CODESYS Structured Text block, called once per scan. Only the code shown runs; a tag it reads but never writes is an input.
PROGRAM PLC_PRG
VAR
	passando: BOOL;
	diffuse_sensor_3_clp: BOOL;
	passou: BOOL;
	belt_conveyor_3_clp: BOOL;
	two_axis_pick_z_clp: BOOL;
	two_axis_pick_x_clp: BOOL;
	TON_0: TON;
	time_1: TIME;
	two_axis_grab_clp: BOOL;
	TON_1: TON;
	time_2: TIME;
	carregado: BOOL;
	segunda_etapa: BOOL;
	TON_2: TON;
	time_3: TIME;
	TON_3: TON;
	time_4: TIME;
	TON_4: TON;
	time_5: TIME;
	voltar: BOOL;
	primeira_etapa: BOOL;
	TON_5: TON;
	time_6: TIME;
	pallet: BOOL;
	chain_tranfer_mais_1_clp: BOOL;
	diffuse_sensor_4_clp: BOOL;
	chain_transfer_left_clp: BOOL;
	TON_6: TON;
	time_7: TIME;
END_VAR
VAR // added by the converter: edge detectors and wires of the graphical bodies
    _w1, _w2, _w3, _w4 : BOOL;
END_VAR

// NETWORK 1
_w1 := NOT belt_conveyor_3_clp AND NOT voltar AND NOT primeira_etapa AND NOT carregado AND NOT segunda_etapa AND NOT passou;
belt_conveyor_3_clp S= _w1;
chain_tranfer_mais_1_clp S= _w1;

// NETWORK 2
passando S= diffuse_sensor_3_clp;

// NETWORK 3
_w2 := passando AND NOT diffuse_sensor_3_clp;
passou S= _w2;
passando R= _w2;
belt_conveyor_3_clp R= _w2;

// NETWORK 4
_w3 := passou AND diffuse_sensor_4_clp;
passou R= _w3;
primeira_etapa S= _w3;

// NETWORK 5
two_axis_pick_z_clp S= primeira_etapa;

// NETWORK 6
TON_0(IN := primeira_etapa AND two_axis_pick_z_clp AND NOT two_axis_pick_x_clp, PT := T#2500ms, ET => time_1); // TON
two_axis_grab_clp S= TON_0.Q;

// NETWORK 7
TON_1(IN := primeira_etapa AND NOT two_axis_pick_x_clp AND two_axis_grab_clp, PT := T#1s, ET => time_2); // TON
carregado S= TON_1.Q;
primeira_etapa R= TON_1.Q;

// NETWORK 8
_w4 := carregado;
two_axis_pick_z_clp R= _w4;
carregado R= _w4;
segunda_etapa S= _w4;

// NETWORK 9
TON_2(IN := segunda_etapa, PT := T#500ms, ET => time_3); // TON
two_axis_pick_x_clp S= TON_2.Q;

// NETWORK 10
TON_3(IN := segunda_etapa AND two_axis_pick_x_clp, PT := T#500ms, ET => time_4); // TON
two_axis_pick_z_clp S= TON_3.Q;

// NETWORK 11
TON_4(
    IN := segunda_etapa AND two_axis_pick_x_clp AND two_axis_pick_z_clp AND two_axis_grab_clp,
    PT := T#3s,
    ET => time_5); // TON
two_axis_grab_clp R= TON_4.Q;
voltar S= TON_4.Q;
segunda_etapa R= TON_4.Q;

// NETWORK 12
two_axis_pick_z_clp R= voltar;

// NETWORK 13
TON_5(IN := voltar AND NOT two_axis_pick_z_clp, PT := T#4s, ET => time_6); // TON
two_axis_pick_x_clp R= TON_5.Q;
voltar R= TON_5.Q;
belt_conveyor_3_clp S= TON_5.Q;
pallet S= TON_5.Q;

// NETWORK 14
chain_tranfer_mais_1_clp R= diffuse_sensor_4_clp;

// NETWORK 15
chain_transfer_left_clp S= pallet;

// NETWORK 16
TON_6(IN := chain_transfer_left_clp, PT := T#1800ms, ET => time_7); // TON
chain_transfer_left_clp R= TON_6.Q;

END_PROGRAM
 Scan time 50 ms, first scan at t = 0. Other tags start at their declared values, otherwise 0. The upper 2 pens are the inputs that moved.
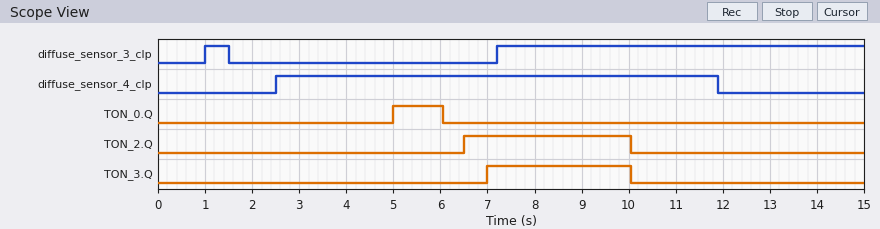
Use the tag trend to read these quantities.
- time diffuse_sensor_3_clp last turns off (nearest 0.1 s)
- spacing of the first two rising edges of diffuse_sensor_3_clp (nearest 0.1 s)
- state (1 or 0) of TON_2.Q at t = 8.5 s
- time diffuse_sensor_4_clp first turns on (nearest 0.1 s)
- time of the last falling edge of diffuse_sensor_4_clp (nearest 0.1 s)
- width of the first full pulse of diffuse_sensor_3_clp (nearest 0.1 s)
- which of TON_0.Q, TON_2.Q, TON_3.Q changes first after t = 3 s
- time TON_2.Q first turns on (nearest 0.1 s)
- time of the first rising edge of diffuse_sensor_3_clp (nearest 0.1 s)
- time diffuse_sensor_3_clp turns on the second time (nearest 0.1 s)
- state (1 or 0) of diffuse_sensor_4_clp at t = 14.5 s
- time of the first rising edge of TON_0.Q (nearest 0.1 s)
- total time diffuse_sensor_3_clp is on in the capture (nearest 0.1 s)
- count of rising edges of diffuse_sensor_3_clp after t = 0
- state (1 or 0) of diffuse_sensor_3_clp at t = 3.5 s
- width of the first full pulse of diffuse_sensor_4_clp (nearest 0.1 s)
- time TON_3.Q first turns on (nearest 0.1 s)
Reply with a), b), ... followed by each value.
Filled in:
a) 1.5 s
b) 6.2 s
c) 1
d) 2.5 s
e) 11.9 s
f) 0.5 s
g) TON_0.Q
h) 6.5 s
i) 1.0 s
j) 7.2 s
k) 0
l) 5.0 s
m) 8.3 s
n) 2
o) 0
p) 9.4 s
q) 7.0 s
